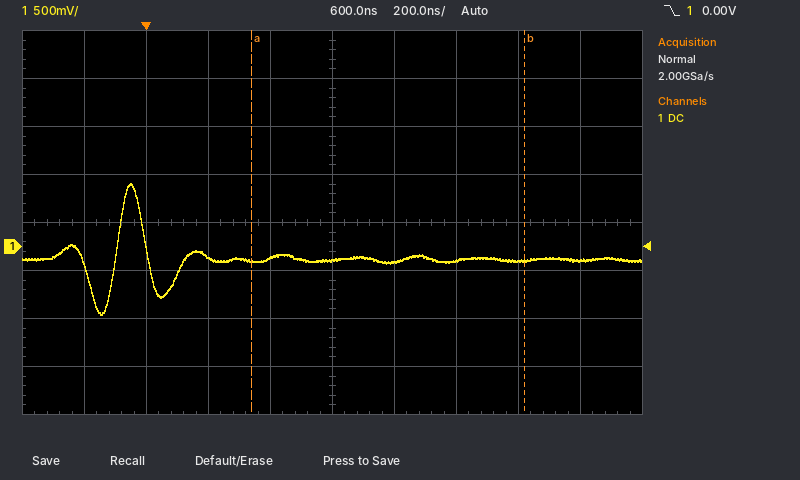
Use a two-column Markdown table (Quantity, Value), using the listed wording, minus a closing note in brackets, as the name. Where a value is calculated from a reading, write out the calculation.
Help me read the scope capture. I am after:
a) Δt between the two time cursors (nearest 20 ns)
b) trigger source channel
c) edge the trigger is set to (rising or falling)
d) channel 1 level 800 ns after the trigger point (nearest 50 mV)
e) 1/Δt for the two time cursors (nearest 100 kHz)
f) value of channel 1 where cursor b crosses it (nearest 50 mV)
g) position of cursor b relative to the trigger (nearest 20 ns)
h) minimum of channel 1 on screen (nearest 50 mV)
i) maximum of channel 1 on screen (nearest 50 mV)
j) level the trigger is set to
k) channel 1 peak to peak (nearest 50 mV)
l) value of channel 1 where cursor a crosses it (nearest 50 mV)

| Quantity | Value |
|---|---|
| Δt between the two time cursors | 880 ns |
| trigger source channel | channel 1 |
| edge the trigger is set to | falling |
| channel 1 level 800 ns after the trigger point | -150 mV |
| 1/Δt for the two time cursors | 1 / 880 ns ≈ 1.1 MHz |
| value of channel 1 where cursor b crosses it | -150 mV |
| position of cursor b relative to the trigger | +1.22 µs |
| minimum of channel 1 on screen | -700 mV |
| maximum of channel 1 on screen | 650 mV |
| level the trigger is set to | 0.00 V |
| channel 1 peak to peak | 650 mV − (-700 mV) = 1.35 V |
| value of channel 1 where cursor a crosses it | -150 mV |
